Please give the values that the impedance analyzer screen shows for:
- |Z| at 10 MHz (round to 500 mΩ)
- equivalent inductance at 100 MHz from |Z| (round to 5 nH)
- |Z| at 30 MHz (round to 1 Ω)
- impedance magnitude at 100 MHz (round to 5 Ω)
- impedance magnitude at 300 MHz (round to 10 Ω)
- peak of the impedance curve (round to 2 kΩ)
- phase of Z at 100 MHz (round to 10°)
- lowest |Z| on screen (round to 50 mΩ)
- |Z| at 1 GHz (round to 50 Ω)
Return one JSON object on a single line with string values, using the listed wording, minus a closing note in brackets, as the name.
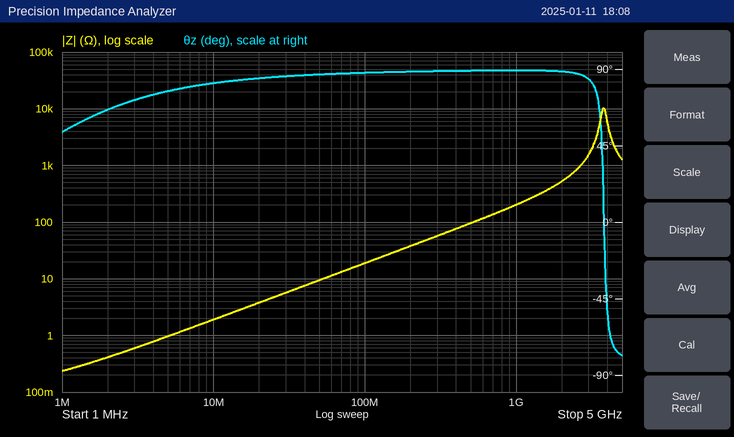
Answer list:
{"|Z| at 10 MHz": "2.0 Ω", "equivalent inductance at 100 MHz from |Z|": "30 nH", "|Z| at 30 MHz": "6 Ω", "impedance magnitude at 100 MHz": "20 Ω", "impedance magnitude at 300 MHz": "60 Ω", "peak of the impedance curve": "10 kΩ", "phase of Z at 100 MHz": "90°", "lowest |Z| on screen": "250 mΩ", "|Z| at 1 GHz": "200 Ω"}
